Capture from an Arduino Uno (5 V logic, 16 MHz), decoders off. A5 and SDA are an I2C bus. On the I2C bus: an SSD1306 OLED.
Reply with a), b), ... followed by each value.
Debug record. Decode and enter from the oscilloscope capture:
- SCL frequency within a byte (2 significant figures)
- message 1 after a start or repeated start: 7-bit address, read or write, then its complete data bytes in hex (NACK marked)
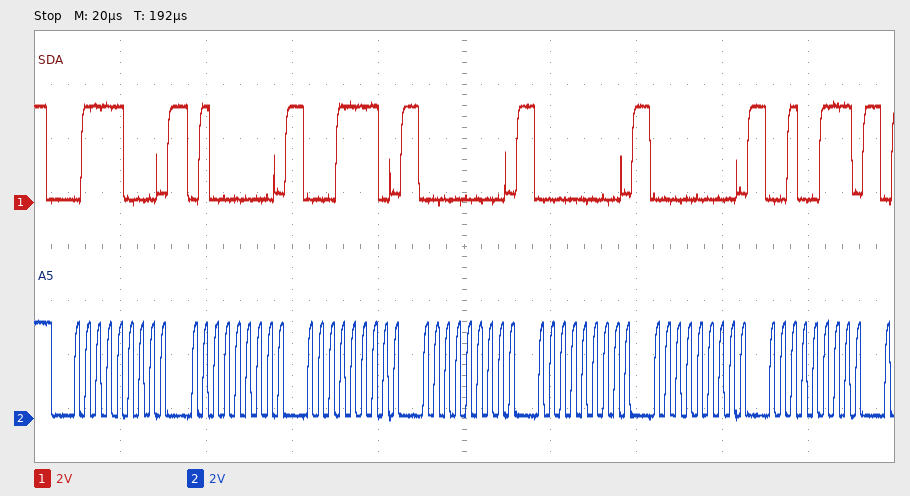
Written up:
a) 400 kHz
b) 0x3C write: 40 1E 00 00 00 27
